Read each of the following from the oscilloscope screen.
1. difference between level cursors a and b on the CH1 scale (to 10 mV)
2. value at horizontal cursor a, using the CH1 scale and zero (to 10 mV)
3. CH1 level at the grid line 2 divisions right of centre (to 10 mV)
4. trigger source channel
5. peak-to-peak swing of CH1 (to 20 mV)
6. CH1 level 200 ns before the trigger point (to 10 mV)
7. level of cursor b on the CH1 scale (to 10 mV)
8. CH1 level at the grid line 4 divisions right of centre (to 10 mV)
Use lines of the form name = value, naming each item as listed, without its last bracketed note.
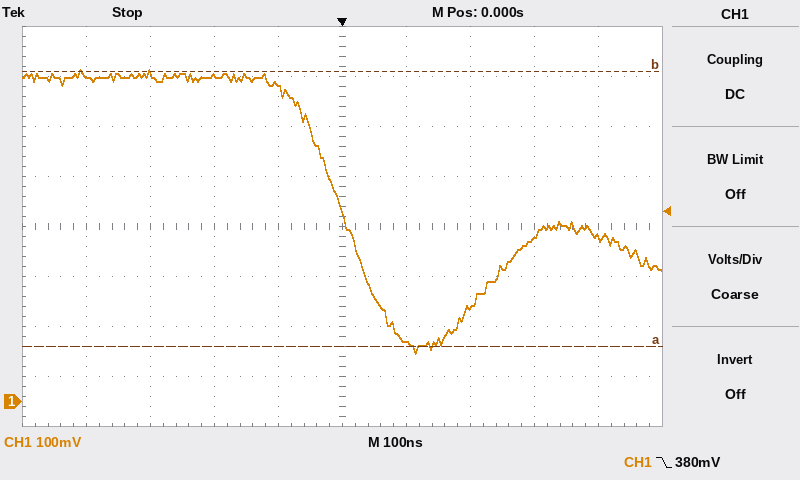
difference between level cursors a and b on the CH1 scale = 550 mV
value at horizontal cursor a, using the CH1 scale and zero = 110 mV
CH1 level at the grid line 2 divisions right of centre = 190 mV
trigger source channel = CH1
peak-to-peak swing of CH1 = 560 mV
CH1 level 200 ns before the trigger point = 650 mV
level of cursor b on the CH1 scale = 660 mV
CH1 level at the grid line 4 divisions right of centre = 330 mV
